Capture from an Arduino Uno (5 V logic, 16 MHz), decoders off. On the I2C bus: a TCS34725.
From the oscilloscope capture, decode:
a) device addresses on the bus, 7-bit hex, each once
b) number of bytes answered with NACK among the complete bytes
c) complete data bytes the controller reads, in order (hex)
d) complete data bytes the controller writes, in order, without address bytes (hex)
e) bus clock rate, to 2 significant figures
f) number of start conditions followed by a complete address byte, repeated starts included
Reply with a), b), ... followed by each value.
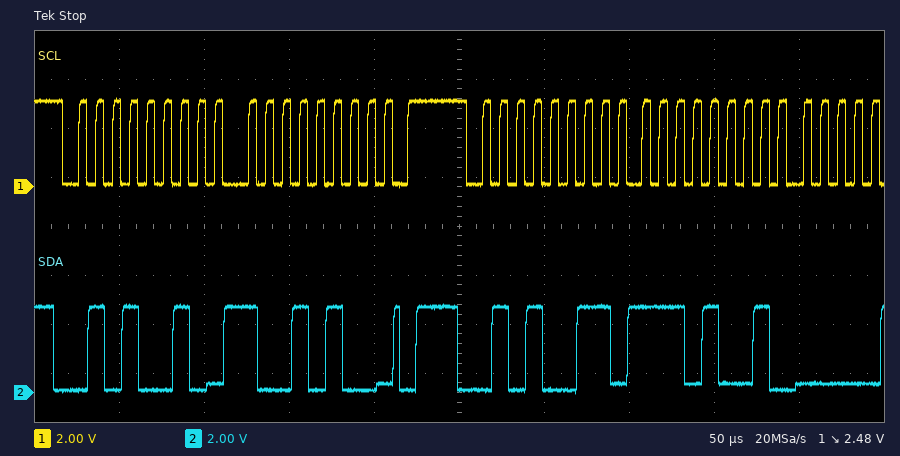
a) 0x29
b) 0
c) E9
d) 94
e) 100 kHz
f) 2
